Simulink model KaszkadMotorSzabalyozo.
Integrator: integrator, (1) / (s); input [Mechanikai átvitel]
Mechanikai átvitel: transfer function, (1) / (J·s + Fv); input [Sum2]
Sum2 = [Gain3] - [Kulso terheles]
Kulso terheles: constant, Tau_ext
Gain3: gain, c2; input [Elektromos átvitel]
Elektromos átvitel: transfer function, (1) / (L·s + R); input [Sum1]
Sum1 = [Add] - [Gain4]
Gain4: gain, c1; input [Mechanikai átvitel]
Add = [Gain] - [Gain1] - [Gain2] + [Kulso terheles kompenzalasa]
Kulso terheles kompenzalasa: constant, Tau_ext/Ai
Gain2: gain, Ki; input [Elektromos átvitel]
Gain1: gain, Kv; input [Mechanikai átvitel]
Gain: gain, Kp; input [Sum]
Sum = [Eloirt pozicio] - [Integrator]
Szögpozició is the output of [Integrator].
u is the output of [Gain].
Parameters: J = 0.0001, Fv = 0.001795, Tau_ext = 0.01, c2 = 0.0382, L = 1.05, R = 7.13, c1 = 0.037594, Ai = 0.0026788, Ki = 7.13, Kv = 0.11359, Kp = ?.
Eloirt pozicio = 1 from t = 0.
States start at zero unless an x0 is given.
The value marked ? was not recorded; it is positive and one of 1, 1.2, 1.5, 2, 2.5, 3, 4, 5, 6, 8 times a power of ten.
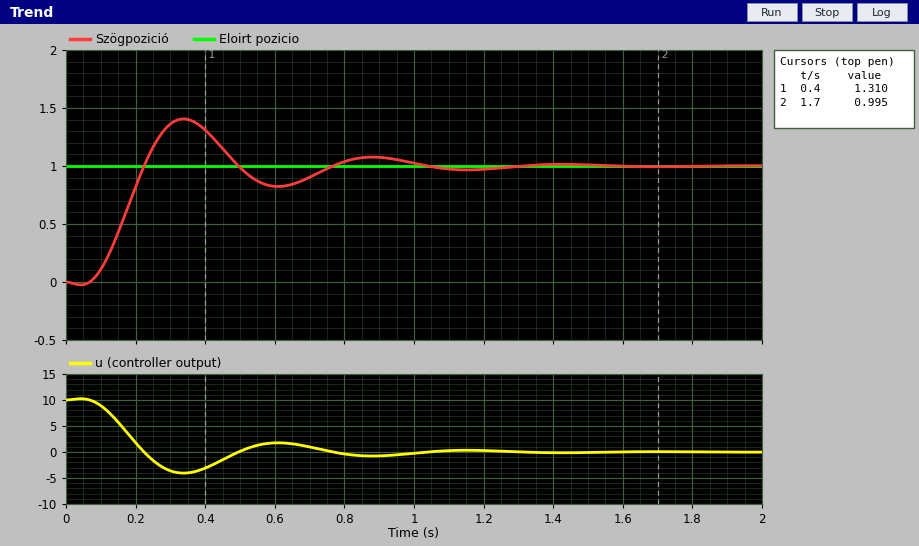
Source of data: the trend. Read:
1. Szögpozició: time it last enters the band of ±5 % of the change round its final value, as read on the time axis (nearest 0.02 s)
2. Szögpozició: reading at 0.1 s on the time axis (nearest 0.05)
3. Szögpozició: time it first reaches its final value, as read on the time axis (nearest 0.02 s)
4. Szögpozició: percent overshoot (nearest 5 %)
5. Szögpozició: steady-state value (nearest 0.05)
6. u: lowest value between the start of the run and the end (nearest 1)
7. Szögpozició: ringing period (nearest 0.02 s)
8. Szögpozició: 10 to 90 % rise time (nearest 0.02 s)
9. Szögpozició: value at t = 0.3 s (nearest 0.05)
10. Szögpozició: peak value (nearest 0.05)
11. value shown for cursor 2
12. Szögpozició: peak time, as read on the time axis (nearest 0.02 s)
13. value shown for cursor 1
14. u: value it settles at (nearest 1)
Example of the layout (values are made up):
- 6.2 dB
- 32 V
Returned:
- 0.96 s
- 0.10
- 0.22 s
- 40 %
- 1.00
- -4
- 0.54 s
- 0.12 s
- 1.35
- 1.40
- 0.995
- 0.34 s
- 1.310
- 0
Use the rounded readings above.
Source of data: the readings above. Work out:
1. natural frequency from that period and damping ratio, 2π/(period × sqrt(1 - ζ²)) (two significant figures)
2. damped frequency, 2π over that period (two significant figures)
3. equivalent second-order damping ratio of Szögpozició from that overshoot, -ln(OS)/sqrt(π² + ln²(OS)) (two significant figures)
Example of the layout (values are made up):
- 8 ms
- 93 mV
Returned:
- 12 rad/s
- 12 rad/s
- 0.28
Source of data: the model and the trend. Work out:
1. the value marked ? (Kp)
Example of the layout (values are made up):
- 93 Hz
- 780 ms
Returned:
- 10
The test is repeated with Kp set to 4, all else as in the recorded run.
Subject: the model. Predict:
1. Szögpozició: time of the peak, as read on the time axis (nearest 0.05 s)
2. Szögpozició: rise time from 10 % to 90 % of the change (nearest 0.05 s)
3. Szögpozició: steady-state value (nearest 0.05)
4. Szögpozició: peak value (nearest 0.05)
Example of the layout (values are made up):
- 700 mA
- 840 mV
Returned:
- 0.60 s
- 0.25 s
- 1.00
- 1.05
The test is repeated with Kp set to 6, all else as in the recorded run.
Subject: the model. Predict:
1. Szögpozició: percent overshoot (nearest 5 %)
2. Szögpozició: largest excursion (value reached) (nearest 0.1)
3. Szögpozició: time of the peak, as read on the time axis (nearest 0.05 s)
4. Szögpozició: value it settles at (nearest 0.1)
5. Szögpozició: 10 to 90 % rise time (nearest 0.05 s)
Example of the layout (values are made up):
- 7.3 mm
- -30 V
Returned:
- 20 %
- 1.2
- 0.45 s
- 1.0
- 0.15 s
